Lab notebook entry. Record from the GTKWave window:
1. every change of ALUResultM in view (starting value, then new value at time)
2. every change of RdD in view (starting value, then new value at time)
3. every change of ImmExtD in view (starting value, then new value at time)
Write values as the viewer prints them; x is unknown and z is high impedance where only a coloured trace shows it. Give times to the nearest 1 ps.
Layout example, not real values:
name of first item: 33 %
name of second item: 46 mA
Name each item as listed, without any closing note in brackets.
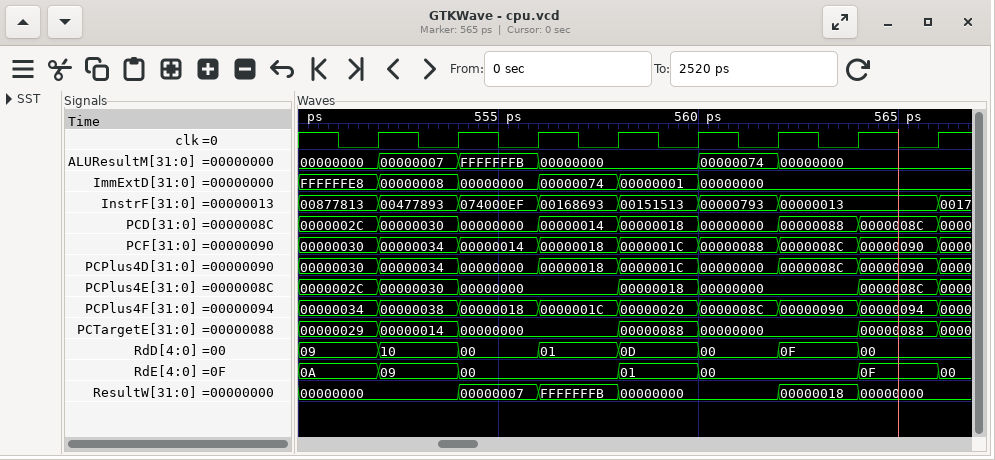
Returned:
every change of ALUResultM in view: 00000000, 00000007 at 552 ps, FFFFFFFB at 554 ps, 00000000 at 556 ps, 00000074 at 560 ps, 00000000 at 562 ps
every change of RdD in view: 09, 10 at 552 ps, 00 at 554 ps, 01 at 556 ps, 0D at 558 ps, 00 at 560 ps, 0F at 562 ps, 00 at 564 ps
every change of ImmExtD in view: FFFFFFE8, 00000008 at 552 ps, 00000000 at 554 ps, 00000074 at 556 ps, 00000001 at 558 ps, 00000000 at 560 ps
